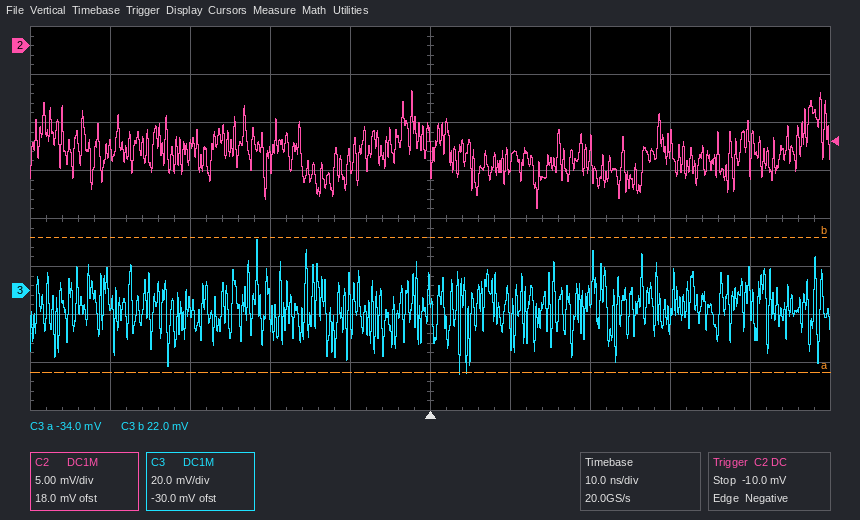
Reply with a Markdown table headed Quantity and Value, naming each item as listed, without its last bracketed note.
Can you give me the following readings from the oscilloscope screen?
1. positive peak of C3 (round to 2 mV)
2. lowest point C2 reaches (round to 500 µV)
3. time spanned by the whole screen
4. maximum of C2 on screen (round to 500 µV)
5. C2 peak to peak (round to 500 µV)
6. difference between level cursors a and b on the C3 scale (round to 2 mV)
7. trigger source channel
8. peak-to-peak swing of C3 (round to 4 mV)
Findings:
| Quantity | Value |
|---|---|
| positive peak of C3 | 22 mV |
| lowest point C2 reaches | -17.0 mV |
| time spanned by the whole screen | 100 ns |
| maximum of C2 on screen | -4.5 mV |
| C2 peak to peak | 12.5 mV |
| difference between level cursors a and b on the C3 scale | 56 mV |
| trigger source channel | C2 |
| peak-to-peak swing of C3 | 56 mV |
